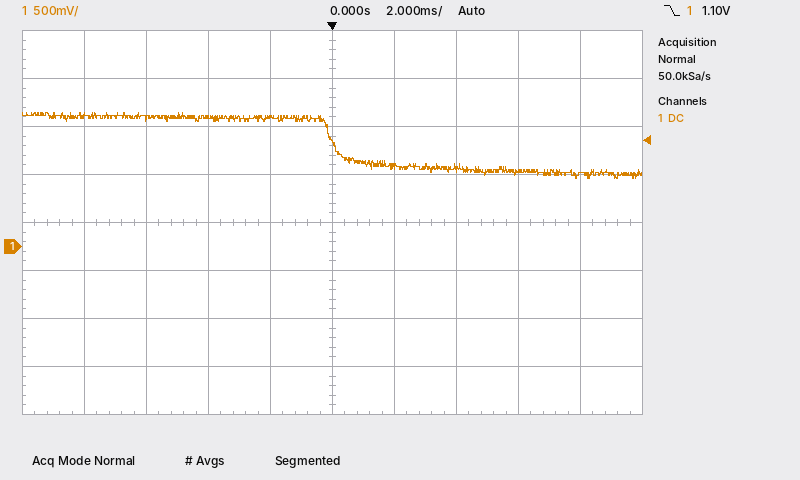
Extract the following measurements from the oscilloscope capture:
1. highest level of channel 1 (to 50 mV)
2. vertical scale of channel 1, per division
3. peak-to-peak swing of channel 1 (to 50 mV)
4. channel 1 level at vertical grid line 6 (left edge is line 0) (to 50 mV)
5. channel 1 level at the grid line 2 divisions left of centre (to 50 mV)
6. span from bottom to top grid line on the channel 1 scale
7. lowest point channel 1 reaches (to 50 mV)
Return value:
1.40 V
500 mV
700 mV
850 mV
1.35 V
4 V
700 mV
